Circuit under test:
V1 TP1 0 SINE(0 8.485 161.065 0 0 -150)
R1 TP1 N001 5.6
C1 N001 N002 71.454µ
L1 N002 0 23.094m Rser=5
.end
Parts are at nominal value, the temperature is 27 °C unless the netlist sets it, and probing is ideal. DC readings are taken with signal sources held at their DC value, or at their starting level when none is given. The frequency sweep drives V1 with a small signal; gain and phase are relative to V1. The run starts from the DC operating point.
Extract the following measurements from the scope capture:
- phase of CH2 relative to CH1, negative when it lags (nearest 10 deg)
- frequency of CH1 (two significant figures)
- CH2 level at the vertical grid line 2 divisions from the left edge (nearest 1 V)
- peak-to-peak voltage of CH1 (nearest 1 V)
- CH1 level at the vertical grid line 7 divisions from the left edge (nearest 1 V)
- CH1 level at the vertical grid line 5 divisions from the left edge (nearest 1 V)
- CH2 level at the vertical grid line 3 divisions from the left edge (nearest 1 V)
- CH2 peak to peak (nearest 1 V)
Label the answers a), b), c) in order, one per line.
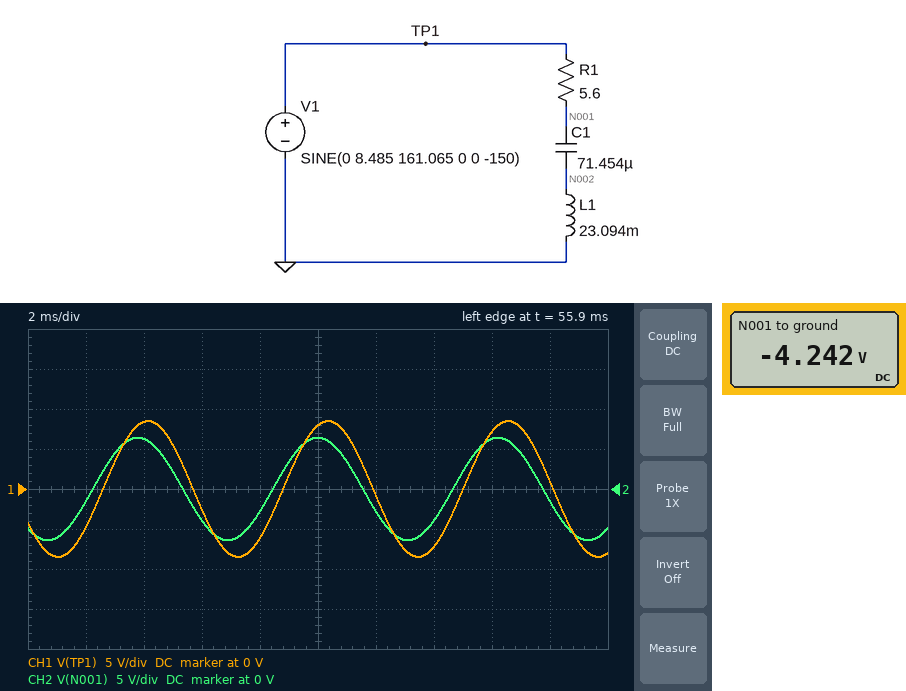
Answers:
a) 20 deg
b) 160 Hz
c) 6 V
d) 17 V
e) -7 V
f) 8 V
g) -4 V
h) 13 V
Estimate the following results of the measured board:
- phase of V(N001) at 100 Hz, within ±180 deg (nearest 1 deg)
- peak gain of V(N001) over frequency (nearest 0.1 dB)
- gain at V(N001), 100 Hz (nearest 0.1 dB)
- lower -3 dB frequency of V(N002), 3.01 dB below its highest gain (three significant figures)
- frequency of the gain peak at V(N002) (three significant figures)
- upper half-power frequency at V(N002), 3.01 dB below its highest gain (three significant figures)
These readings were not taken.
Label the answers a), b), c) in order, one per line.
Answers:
a) -21 deg
b) 0 dB
c) -3.1 dB
d) 104 Hz
e) 135 Hz
f) 232 Hz
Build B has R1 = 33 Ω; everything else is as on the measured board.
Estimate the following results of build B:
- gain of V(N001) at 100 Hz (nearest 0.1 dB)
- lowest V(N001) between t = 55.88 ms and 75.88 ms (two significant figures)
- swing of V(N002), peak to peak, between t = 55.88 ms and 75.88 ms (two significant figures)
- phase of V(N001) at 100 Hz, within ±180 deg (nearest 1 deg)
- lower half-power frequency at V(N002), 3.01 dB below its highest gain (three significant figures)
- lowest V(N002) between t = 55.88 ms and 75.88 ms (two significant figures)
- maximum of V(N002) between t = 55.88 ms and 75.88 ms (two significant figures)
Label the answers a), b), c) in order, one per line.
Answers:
a) -12.5 dB
b) -2.3 V
c) 10 V
d) -46 deg
e) 203 Hz
f) -5.2 V
g) 5.2 V
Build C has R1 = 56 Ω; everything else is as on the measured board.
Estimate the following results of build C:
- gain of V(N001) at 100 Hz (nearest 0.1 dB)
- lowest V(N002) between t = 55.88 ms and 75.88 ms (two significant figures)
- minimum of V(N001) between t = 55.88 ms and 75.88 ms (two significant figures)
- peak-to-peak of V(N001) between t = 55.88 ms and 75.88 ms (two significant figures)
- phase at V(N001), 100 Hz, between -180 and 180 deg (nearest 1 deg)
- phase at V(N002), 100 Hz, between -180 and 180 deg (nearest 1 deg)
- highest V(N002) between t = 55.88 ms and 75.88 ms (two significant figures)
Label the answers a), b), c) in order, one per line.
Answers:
a) -16.5 dB
b) -3.3 V
c) -1.5 V
d) 3.0 V
e) -50 deg
f) 78 deg
g) 3.3 V
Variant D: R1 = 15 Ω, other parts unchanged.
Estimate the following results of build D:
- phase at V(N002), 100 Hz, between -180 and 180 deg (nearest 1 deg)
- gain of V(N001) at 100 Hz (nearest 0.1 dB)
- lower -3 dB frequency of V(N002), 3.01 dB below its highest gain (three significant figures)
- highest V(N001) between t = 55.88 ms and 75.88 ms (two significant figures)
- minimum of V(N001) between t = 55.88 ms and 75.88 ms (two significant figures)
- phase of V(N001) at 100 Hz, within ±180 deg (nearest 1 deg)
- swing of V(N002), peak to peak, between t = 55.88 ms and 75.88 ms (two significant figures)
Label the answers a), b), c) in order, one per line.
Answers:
a) 92 deg
b) -7.3 dB
c) 106 Hz
d) 4.1 V
e) -4.1 V
f) -36 deg
g) 18 V
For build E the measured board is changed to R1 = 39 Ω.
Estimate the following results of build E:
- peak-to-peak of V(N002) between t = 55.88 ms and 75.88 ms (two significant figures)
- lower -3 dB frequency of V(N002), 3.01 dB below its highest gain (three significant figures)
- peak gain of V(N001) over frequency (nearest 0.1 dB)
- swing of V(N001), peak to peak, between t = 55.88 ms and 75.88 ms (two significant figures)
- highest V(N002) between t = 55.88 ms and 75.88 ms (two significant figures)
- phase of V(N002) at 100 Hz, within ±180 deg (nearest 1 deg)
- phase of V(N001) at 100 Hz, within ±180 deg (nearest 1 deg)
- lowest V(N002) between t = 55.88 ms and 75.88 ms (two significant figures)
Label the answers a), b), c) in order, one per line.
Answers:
a) 9.0 V
b) 250 Hz
c) 0 dB
d) 4.1 V
e) 4.5 V
f) 81 deg
g) -47 deg
h) -4.5 V
